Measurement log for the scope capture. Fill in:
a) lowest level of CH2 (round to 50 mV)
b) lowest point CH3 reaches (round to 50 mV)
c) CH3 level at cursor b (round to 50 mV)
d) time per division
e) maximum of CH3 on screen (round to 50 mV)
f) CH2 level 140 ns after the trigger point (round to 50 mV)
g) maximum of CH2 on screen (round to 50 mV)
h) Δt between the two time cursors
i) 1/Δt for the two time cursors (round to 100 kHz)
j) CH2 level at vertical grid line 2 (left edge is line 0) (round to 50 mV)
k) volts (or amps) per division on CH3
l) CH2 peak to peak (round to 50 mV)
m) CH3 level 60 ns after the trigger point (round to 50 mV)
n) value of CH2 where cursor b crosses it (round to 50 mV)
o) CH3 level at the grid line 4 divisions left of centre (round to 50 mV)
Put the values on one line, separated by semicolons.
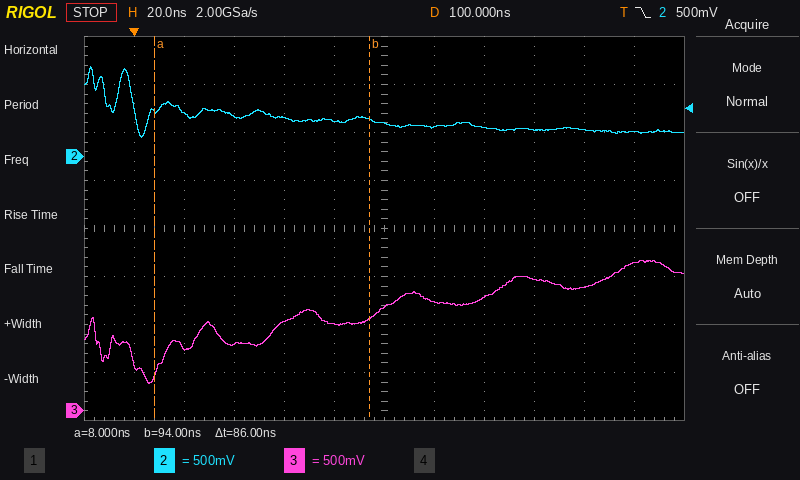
200 mV; 300 mV; 950 mV; 20 ns; 1.55 V; 300 mV; 950 mV; 86 ns; 11.6 MHz; 450 mV; 500 mV; 750 mV; 950 mV; 400 mV; 650 mV
